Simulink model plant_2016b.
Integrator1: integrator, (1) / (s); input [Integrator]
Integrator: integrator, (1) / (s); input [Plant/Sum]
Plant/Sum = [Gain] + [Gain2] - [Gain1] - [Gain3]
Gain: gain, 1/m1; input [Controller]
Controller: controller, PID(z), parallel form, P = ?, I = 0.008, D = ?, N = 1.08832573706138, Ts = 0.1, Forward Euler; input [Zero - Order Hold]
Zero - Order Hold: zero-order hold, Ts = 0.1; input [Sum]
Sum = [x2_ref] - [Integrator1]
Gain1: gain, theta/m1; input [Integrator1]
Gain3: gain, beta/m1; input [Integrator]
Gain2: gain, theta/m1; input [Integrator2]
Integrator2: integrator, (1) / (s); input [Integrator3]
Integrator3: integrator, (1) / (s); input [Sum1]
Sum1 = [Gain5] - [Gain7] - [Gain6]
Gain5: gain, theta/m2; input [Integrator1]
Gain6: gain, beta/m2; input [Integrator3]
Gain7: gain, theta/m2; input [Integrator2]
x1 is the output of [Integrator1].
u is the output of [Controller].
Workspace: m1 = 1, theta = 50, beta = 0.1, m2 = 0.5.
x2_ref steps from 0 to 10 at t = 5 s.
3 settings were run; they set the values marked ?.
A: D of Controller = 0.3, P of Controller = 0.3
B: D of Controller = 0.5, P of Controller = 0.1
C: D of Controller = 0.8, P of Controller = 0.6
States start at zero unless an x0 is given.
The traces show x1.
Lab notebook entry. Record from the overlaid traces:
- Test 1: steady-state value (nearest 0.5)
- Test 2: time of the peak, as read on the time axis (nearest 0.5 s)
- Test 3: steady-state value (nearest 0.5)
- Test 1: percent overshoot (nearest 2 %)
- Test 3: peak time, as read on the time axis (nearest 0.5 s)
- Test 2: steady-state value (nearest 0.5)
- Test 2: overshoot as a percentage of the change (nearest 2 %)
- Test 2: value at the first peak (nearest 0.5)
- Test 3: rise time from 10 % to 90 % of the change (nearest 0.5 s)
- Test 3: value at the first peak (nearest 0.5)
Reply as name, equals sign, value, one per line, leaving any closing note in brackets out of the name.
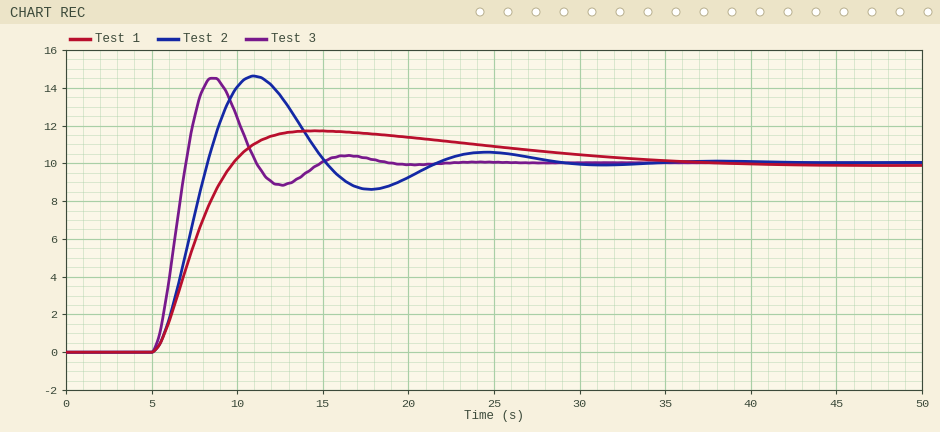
Test 1: steady-state value = 10.0
Test 2: time of the peak, as read on the time axis = 11.0 s
Test 3: steady-state value = 10.0
Test 1: percent overshoot = 18 %
Test 3: peak time, as read on the time axis = 8.5 s
Test 2: steady-state value = 10.0
Test 2: overshoot as a percentage of the change = 46 %
Test 2: value at the first peak = 14.5
Test 3: rise time from 10 % to 90 % of the change = 1.5 s
Test 3: value at the first peak = 14.5
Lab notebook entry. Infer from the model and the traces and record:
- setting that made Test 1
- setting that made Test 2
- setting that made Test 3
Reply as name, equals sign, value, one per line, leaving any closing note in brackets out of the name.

setting that made Test 1 = B
setting that made Test 2 = A
setting that made Test 3 = C
